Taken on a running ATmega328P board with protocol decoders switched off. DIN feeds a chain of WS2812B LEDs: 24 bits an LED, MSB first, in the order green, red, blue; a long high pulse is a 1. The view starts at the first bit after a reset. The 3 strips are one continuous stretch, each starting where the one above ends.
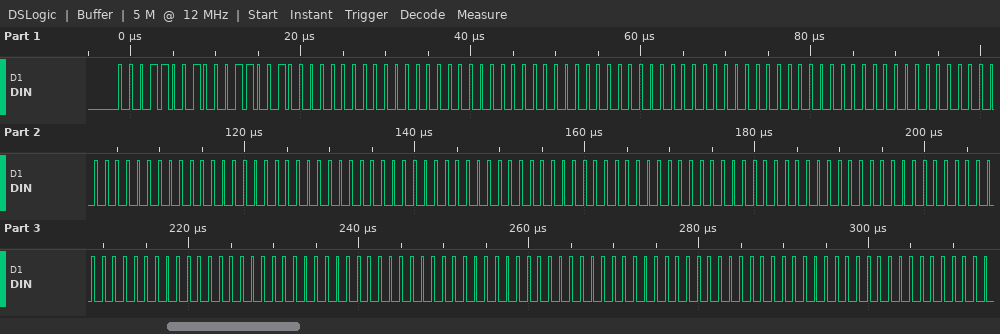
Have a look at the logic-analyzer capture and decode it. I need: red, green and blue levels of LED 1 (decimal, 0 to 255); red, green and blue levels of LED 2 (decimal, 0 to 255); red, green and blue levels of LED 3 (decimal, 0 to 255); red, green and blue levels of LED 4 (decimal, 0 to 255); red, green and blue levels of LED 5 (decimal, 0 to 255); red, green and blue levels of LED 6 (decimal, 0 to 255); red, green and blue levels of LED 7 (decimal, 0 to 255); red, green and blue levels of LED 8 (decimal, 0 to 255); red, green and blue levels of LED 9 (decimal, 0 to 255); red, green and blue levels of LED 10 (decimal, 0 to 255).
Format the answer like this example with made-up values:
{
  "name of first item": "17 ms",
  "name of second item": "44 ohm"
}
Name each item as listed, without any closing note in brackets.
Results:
{
  "red, green and blue levels of LED 1": "25, 25, 0",
  "red, green and blue levels of LED 2": "0, 0, 0",
  "red, green and blue levels of LED 3": "0, 0, 0",
  "red, green and blue levels of LED 4": "0, 0, 0",
  "red, green and blue levels of LED 5": "0, 0, 0",
  "red, green and blue levels of LED 6": "0, 0, 0",
  "red, green and blue levels of LED 7": "0, 0, 0",
  "red, green and blue levels of LED 8": "0, 0, 0",
  "red, green and blue levels of LED 9": "0, 0, 0",
  "red, green and blue levels of LED 10": "0, 0, 0"
}
